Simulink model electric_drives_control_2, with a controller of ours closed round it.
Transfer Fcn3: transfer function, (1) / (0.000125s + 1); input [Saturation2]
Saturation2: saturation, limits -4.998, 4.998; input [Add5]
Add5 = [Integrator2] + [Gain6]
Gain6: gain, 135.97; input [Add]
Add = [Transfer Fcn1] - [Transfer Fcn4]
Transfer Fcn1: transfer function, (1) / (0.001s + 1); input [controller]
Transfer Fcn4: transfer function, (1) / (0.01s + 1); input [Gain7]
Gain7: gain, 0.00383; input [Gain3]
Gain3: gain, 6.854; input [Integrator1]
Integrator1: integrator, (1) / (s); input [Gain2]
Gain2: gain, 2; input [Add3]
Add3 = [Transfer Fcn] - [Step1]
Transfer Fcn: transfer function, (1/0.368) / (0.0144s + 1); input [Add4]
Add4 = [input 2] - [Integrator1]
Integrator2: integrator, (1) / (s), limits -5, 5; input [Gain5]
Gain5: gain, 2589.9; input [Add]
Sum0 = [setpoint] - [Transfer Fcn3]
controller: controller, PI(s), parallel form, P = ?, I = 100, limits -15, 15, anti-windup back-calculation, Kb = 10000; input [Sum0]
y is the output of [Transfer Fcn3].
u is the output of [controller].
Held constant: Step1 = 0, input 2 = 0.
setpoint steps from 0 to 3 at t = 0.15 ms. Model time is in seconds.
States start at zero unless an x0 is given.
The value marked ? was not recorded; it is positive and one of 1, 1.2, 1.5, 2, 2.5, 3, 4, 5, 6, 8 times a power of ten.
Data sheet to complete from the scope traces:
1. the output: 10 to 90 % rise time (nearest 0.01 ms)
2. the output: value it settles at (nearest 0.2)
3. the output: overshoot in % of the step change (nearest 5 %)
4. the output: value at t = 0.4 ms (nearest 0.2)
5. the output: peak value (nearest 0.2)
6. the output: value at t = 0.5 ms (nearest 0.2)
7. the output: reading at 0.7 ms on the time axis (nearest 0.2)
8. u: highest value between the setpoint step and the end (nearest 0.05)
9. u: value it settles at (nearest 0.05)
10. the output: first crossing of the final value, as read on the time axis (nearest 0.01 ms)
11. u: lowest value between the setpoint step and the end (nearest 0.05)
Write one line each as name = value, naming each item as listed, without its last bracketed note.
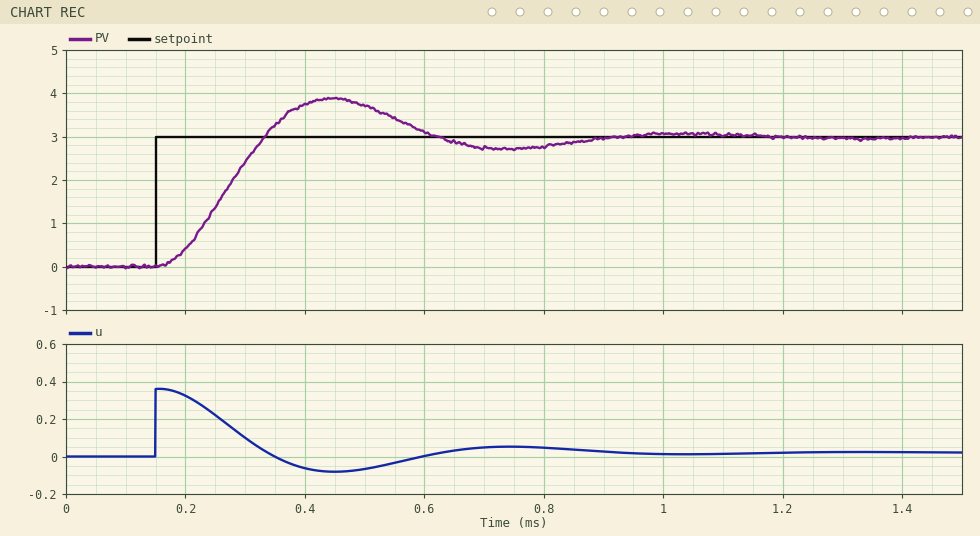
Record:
the output: 10 to 90 % rise time = 0.12 ms
the output: value it settles at = 3.0
the output: overshoot in % of the step change = 30 %
the output: value at t = 0.4 ms = 3.8
the output: peak value = 3.8
the output: value at t = 0.5 ms = 3.8
the output: reading at 0.7 ms on the time axis = 2.8
u: highest value between the setpoint step and the end = 0.35
u: value it settles at = 0.00
the output: first crossing of the final value, as read on the time axis = 0.33 ms
u: lowest value between the setpoint step and the end = -0.10
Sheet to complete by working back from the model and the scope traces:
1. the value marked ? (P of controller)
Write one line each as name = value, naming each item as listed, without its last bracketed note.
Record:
the value marked ? = 0.12
